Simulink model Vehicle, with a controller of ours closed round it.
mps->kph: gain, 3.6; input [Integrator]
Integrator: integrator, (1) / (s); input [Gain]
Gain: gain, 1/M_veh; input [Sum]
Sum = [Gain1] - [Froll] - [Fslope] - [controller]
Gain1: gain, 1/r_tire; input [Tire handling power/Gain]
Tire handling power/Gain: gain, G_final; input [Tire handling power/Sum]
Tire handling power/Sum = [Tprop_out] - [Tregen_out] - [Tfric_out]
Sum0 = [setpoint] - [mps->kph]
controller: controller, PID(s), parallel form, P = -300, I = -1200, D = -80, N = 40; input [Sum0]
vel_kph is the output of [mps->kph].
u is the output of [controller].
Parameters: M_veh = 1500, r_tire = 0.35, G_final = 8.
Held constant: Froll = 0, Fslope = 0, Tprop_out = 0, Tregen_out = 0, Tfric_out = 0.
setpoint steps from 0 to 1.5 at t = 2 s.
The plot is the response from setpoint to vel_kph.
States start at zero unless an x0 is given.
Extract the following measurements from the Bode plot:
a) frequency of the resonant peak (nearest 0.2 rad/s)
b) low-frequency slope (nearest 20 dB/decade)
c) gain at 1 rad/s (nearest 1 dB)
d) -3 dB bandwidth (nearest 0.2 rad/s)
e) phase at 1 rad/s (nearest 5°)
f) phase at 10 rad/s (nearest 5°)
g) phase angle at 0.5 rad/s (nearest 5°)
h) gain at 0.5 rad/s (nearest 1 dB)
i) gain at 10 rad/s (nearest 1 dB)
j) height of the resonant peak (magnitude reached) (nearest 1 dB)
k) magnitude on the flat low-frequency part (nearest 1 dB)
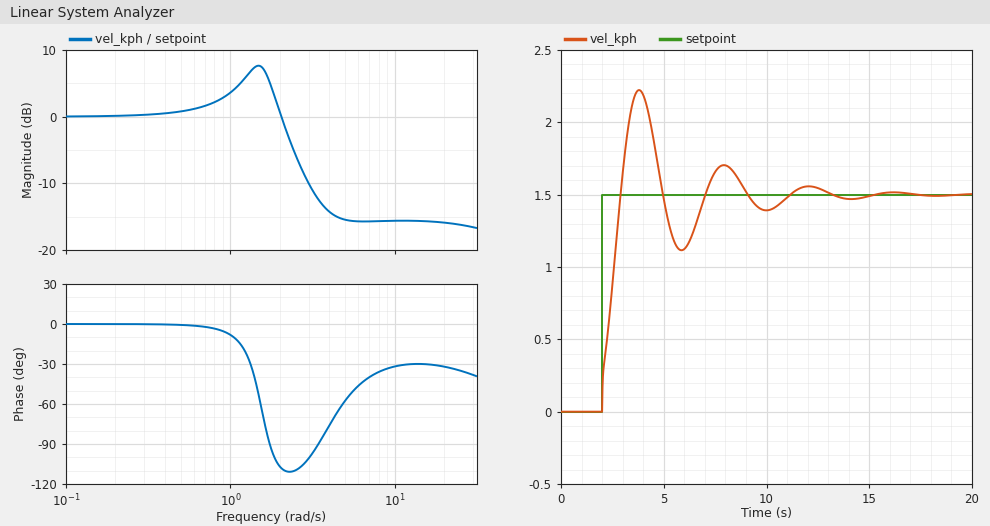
1.4 rad/s
0 dB/decade
4 dB
2.2 rad/s
-10°
-30°
0°
1 dB
-16 dB
8 dB
0 dB
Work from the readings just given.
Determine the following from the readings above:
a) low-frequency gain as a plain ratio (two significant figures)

1.0
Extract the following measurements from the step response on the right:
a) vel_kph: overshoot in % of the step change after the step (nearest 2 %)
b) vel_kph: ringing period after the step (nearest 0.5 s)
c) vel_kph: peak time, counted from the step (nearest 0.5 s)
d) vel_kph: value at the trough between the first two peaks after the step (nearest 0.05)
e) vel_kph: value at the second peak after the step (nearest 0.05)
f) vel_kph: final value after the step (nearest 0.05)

48 %
4.0 s
2.0 s
1.10
1.70
1.50
